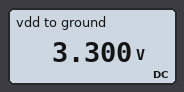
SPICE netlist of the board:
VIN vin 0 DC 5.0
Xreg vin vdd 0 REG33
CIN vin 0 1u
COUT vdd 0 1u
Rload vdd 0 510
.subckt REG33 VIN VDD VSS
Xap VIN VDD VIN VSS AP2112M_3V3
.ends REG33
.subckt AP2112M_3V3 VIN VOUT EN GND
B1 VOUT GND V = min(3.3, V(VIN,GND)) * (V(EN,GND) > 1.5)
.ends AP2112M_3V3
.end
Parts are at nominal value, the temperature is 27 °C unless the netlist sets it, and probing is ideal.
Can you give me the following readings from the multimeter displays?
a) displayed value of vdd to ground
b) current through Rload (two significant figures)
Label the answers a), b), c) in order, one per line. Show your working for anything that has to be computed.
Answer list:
a) 3.300 V
b) (3.3 V) / 510 Ω = 6.5 mA
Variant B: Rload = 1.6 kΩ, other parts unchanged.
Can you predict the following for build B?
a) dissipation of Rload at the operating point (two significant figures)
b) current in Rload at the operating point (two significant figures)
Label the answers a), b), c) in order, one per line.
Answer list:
a) 6.8 mW
b) 2.1 mA
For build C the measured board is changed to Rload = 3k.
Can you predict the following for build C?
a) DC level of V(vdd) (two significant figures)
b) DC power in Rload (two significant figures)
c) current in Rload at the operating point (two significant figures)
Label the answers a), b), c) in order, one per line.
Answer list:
a) 3.3 V
b) 3.6 mW
c) 1.1 mA
